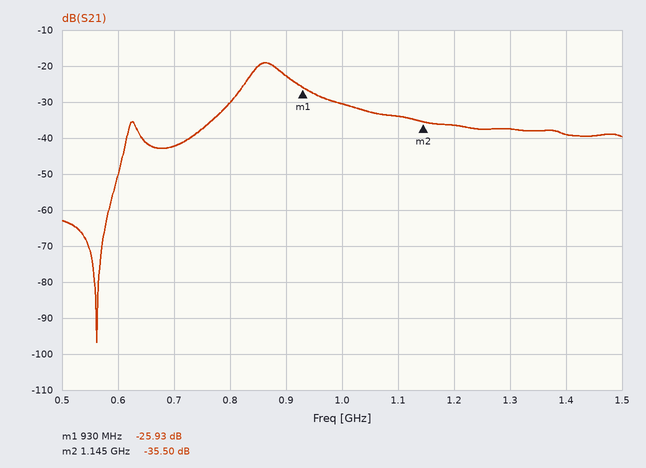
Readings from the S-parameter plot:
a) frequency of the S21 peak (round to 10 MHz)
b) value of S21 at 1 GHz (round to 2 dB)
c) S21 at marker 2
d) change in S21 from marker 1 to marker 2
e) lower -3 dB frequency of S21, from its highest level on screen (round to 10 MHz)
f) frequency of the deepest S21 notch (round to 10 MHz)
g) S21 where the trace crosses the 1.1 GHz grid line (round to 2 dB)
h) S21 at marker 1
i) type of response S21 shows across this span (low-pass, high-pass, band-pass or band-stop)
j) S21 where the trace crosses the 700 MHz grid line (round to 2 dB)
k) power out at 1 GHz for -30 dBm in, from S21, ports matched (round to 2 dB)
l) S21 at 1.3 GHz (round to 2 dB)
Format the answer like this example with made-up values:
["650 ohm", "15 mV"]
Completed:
["860 MHz", "-30 dB", "-35.50 dB", "-9.57 dB", "840 MHz", "560 MHz", "-34 dB", "-25.93 dB", "band-pass", "-42 dB", "-60 dBm", "-38 dB"]
